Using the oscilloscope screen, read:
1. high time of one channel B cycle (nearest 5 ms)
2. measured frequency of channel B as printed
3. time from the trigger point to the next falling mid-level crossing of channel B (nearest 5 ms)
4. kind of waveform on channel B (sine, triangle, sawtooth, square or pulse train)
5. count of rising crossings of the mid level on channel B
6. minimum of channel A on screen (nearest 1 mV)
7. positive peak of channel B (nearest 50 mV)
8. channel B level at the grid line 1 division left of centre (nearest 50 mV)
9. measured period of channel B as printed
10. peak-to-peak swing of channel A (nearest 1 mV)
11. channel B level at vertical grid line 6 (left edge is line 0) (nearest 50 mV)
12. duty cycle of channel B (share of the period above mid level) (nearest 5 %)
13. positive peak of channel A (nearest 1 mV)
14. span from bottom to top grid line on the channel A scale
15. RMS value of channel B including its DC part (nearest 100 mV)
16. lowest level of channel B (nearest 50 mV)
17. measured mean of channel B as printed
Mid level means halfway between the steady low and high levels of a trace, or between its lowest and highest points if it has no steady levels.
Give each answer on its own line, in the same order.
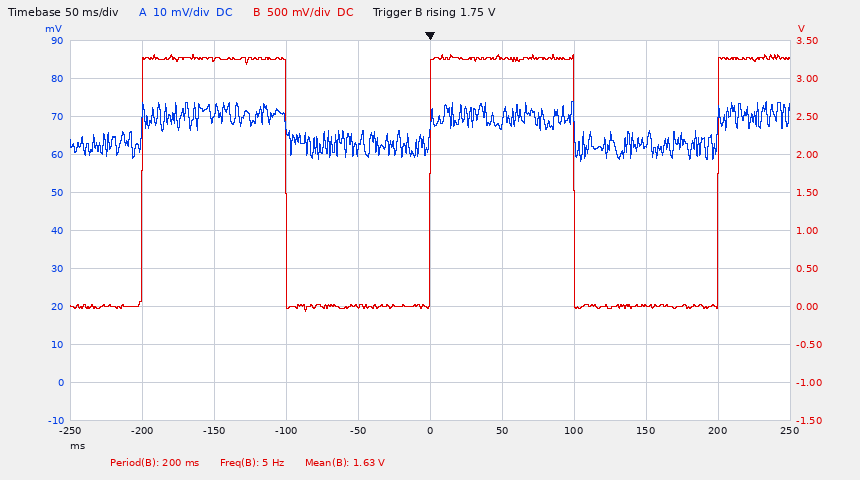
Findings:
100 ms
5 Hz
100 ms
square
3
58 mV
3.30 V
0 mV
200 ms
16 mV
3.25 V
50 %
74 mV
100 mV
2.3 V
-50 mV
1.63 V
